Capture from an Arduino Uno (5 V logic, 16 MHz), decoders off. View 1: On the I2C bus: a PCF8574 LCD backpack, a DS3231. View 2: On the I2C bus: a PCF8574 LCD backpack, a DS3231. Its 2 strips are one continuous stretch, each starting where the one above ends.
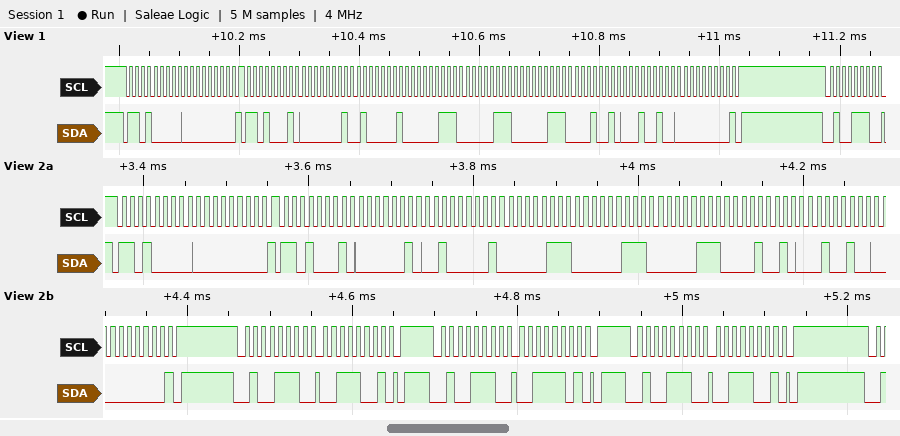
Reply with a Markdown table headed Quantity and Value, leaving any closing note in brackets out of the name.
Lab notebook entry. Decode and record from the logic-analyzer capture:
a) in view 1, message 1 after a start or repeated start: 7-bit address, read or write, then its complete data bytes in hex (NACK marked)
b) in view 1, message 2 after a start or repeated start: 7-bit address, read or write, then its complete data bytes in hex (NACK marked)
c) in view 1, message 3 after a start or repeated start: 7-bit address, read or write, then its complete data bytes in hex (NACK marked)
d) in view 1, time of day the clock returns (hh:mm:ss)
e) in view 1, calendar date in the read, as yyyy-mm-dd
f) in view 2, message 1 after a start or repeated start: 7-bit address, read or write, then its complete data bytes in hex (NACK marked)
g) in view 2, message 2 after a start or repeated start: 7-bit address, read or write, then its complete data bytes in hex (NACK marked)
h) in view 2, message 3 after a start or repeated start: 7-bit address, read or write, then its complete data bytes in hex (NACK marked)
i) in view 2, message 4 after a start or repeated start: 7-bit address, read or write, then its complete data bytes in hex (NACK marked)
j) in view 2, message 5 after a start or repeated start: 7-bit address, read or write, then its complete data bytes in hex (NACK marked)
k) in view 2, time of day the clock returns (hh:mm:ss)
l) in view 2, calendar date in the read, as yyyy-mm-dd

| Quantity | Value |
|---|---|
| in view 1, message 1 after a start or repeated start: 7-bit address, read or write, then its complete data bytes in hex | 0x68 write: 00 |
| in view 1, message 2 after a start or repeated start: 7-bit address, read or write, then its complete data bytes in hex | 0x68 read: 01 41 07 07 07 12 24 00 NACK |
| in view 1, message 3 after a start or repeated start: 7-bit address, read or write, then its complete data bytes in hex | 0x27 write |
| in view 1, time of day the clock returns | 07:41:01 |
| in view 1, calendar date in the read, as yyyy-mm-dd | 2024-12-07 |
| in view 2, message 1 after a start or repeated start: 7-bit address, read or write, then its complete data bytes in hex | 0x68 write: 00 |
| in view 2, message 2 after a start or repeated start: 7-bit address, read or write, then its complete data bytes in hex | 0x68 read: 02 41 07 07 07 12 24 00 NACK |
| in view 2, message 3 after a start or repeated start: 7-bit address, read or write, then its complete data bytes in hex | 0x27 write: 39 |
| in view 2, message 4 after a start or repeated start: 7-bit address, read or write, then its complete data bytes in hex | 0x27 write: 3D |
| in view 2, message 5 after a start or repeated start: 7-bit address, read or write, then its complete data bytes in hex | 0x27 write: 39 |
| in view 2, time of day the clock returns | 07:41:02 |
| in view 2, calendar date in the read, as yyyy-mm-dd | 2024-12-07 |
